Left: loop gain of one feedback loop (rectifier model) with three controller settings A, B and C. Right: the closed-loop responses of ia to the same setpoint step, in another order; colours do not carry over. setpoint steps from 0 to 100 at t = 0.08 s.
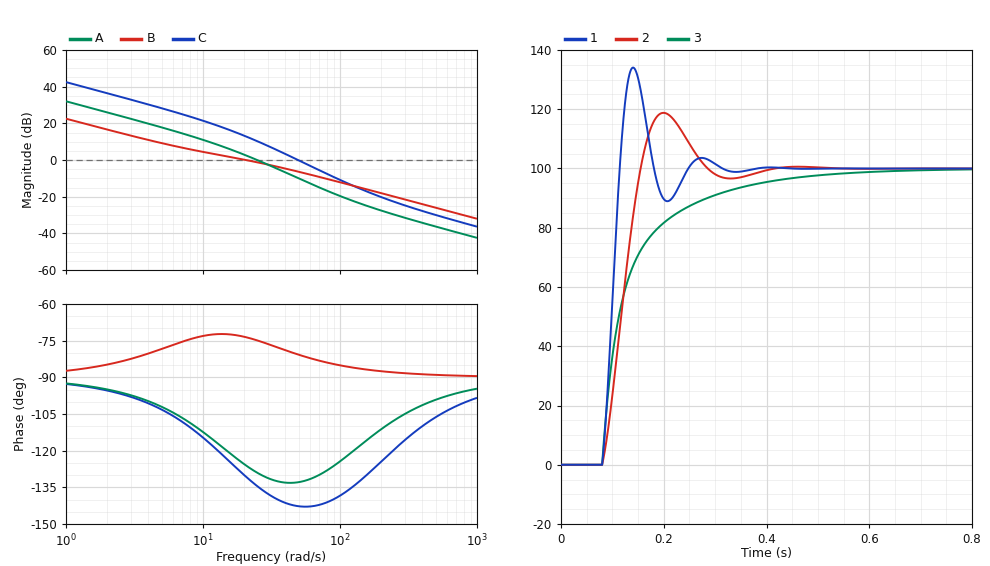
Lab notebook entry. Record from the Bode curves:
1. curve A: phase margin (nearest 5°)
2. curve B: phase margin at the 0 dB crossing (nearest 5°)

50°
105°
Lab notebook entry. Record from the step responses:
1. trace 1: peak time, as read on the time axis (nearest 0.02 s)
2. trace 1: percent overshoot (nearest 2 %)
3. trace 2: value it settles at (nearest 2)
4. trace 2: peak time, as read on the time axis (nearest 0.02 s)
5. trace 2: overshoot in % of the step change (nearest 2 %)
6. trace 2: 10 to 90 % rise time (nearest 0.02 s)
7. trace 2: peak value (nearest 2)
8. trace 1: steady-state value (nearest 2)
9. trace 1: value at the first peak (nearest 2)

0.14 s
34 %
100
0.20 s
18 %
0.06 s
118
100
134
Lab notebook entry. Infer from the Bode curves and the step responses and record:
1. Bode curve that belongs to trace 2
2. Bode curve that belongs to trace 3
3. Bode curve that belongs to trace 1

A
B
C
